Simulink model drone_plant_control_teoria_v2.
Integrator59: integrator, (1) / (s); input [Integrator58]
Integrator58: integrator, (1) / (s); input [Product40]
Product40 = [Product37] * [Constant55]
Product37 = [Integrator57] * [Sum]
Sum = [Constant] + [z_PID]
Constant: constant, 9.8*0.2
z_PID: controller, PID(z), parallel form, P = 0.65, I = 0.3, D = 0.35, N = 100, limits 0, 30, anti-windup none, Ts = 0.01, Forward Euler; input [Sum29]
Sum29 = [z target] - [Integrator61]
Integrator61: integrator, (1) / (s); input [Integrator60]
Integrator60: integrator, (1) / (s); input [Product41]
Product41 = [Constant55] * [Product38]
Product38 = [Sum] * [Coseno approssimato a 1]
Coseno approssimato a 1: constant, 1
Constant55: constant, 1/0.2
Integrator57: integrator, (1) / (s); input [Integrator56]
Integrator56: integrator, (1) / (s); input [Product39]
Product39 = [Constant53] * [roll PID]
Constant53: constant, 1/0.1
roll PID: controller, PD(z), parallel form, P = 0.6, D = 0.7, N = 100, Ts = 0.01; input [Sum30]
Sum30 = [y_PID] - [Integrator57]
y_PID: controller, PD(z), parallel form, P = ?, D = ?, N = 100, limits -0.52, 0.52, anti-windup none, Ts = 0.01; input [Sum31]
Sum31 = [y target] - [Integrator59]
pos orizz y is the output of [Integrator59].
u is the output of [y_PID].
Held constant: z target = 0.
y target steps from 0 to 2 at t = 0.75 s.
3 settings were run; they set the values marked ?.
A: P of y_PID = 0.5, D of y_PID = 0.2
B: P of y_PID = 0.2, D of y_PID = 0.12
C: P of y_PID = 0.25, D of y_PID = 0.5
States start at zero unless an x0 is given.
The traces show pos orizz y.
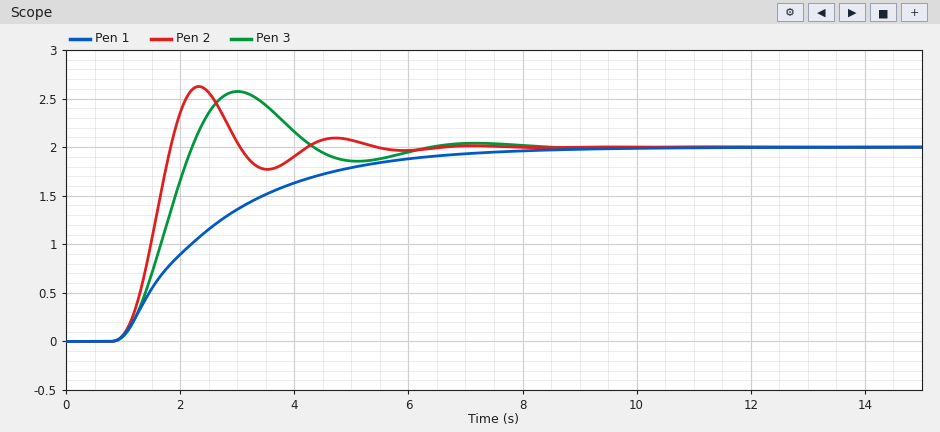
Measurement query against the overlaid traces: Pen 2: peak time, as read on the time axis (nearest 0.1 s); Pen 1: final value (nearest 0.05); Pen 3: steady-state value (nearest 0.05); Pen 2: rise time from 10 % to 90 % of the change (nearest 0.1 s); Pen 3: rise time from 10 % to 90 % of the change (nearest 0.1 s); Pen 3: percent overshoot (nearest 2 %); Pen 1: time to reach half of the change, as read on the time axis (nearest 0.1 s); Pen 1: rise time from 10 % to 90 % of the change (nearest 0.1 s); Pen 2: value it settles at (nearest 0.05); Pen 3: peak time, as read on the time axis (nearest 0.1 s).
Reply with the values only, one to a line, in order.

2.3 s
2.00
2.00
0.6 s
0.9 s
28 %
2.2 s
3.9 s
2.00
3.0 s
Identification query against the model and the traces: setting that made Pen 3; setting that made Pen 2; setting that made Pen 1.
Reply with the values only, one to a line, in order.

B
A
C
